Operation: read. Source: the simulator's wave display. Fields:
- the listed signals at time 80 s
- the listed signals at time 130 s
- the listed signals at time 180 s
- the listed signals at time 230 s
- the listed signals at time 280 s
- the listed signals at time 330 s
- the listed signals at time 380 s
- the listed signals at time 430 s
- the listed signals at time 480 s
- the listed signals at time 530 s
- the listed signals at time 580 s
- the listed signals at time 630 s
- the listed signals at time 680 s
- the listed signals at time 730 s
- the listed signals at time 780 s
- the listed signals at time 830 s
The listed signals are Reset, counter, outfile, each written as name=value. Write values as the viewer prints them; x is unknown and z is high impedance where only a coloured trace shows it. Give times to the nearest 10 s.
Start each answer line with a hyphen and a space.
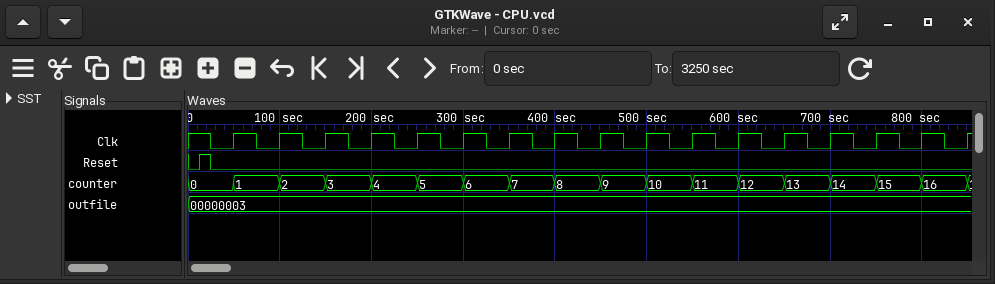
- Reset=0, counter=1, outfile=00000003
- Reset=0, counter=2, outfile=00000003
- Reset=0, counter=3, outfile=00000003
- Reset=0, counter=4, outfile=00000003
- Reset=0, counter=5, outfile=00000003
- Reset=0, counter=6, outfile=00000003
- Reset=0, counter=7, outfile=00000003
- Reset=0, counter=8, outfile=00000003
- Reset=0, counter=9, outfile=00000003
- Reset=0, counter=10, outfile=00000003
- Reset=0, counter=11, outfile=00000003
- Reset=0, counter=12, outfile=00000003
- Reset=0, counter=13, outfile=00000003
- Reset=0, counter=14, outfile=00000003
- Reset=0, counter=15, outfile=00000003
- Reset=0, counter=16, outfile=00000003
